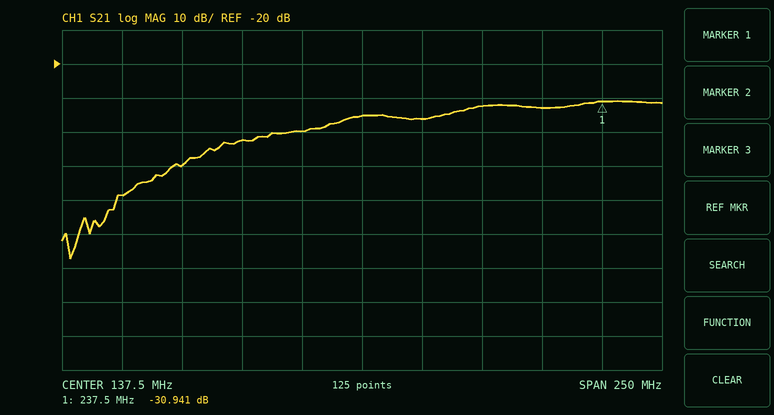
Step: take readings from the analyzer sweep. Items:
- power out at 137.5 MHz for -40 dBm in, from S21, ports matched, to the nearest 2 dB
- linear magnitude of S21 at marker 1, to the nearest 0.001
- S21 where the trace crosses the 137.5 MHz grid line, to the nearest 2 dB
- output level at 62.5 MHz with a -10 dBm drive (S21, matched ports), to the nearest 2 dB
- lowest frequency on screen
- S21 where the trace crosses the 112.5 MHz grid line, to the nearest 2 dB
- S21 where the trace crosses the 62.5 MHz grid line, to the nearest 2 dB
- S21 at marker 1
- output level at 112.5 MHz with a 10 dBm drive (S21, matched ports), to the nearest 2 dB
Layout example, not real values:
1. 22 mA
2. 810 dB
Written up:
1. -76 dBm
2. 0.028
3. -36 dB
4. -60 dBm
5. 12.5 MHz
6. -40 dB
7. -50 dB
8. -30.941 dB
9. -30 dBm
